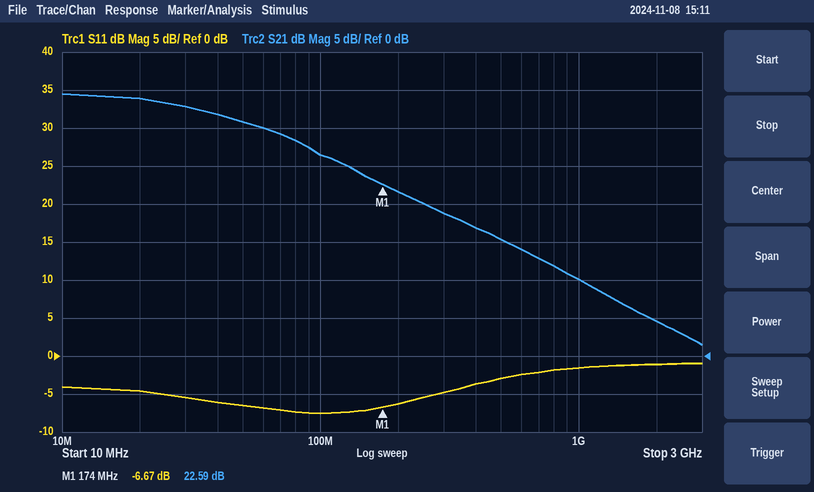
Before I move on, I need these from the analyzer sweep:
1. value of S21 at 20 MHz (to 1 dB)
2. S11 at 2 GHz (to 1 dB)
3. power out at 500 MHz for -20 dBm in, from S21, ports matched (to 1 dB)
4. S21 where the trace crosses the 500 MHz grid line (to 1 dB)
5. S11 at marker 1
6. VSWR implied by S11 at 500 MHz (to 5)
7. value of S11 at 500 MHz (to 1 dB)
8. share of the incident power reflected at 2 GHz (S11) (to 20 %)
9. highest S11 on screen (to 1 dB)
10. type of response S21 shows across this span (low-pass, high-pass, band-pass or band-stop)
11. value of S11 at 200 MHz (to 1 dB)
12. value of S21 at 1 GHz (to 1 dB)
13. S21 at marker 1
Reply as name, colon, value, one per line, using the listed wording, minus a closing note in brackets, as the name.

value of S21 at 20 MHz: 34 dB
S11 at 2 GHz: -1 dB
power out at 500 MHz for -20 dBm in, from S21, ports matched: -5 dBm
S21 where the trace crosses the 500 MHz grid line: 15 dB
S11 at marker 1: -6.67 dB
VSWR implied by S11 at 500 MHz: 5
value of S11 at 500 MHz: -3 dB
share of the incident power reflected at 2 GHz (S11): 80 %
highest S11 on screen: -1 dB
type of response S21 shows across this span: low-pass
value of S11 at 200 MHz: -6 dB
value of S21 at 1 GHz: 10 dB
S21 at marker 1: 22.59 dB
